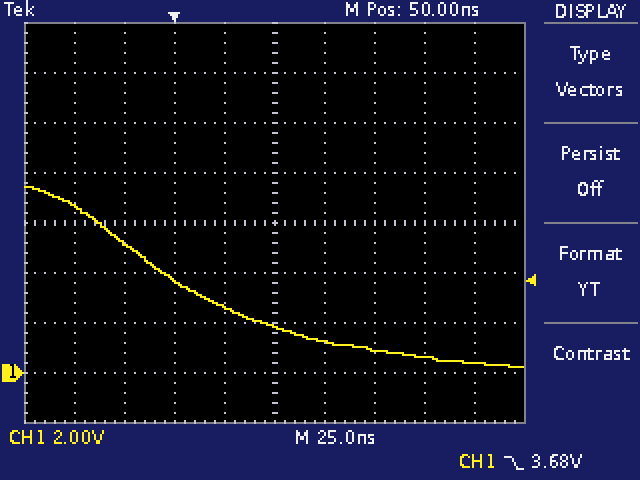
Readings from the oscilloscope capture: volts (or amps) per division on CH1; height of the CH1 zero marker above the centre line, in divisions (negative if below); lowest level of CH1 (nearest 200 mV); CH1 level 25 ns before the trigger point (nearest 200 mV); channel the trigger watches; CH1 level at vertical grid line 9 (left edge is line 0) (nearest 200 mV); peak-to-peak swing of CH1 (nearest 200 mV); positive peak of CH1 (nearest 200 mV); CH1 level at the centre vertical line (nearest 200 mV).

2 V
-3.0 div
200 mV
5.2 V
CH1
400 mV
7.2 V
7.4 V
1.8 V
